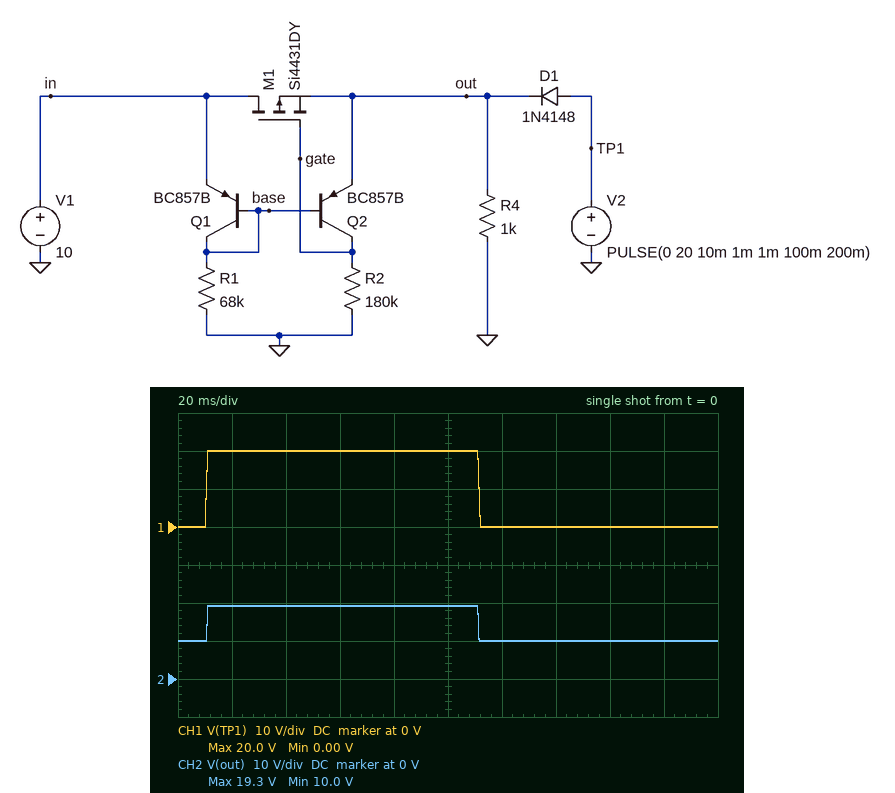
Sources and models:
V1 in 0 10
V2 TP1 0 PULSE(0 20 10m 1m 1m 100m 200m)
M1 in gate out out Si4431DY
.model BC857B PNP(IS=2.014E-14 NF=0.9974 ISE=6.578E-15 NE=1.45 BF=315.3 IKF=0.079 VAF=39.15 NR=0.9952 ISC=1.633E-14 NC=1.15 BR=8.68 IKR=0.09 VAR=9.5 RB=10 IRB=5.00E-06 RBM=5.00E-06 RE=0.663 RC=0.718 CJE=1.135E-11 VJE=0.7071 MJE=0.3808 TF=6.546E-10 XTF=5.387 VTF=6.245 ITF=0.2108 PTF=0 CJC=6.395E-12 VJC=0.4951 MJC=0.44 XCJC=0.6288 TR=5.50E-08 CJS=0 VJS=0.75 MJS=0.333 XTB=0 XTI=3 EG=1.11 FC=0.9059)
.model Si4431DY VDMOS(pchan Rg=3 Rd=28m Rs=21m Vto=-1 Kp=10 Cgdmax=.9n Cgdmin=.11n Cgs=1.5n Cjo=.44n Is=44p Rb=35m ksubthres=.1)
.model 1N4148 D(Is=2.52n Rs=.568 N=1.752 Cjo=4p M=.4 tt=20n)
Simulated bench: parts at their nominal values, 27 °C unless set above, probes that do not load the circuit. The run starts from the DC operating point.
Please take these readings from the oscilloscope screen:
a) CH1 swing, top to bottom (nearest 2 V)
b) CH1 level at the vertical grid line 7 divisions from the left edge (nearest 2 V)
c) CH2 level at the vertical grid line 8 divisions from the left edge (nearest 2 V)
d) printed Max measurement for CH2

20 V
0 V
10 V
19.3 V
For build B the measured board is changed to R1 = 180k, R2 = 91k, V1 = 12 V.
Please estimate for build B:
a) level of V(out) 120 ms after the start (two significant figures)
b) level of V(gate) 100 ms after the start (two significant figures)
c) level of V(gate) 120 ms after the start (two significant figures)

12 V
19 V
6.3 V
